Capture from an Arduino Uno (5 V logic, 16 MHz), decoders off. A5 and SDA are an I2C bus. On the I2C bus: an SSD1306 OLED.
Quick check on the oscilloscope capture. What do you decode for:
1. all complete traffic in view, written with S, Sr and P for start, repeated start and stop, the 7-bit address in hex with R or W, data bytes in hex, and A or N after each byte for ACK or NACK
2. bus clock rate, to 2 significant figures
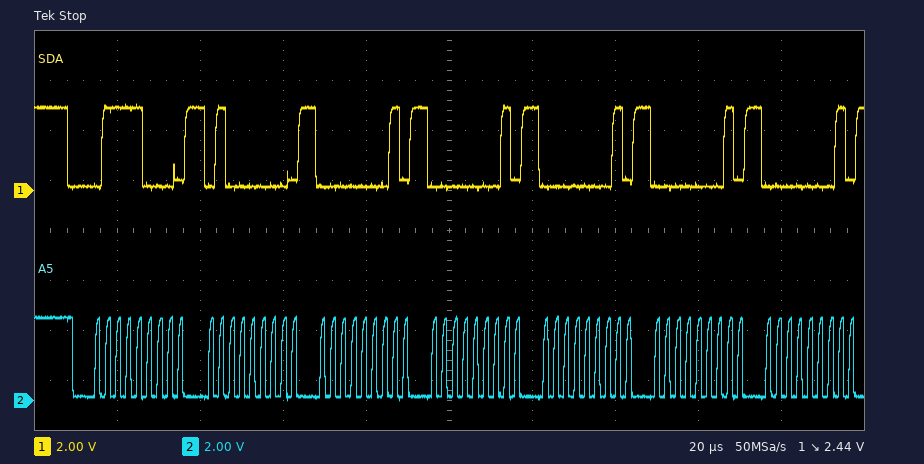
S 3CW A 40 A 01 A 01 A 01 A 01 A 01 A
400 kHz
